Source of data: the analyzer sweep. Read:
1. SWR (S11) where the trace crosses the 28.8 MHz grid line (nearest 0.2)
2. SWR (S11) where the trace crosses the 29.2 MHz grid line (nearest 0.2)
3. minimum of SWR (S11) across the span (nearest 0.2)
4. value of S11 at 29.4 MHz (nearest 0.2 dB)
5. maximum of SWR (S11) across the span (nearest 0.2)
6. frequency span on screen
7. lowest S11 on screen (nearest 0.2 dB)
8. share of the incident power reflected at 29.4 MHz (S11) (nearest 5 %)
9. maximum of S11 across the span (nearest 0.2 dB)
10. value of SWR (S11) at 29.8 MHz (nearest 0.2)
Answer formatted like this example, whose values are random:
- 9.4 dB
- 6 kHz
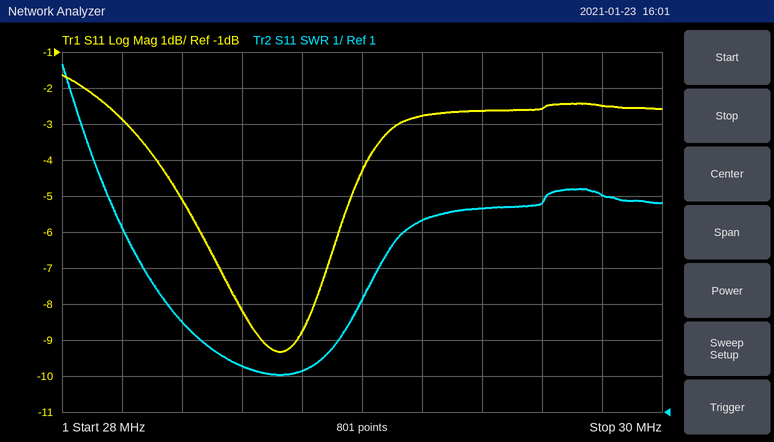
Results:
- 2.2
- 6.4
- 2.0
- -2.6 dB
- 10.6
- 2 MHz
- -9.4 dB
- 55 %
- -1.6 dB
- 7.0
